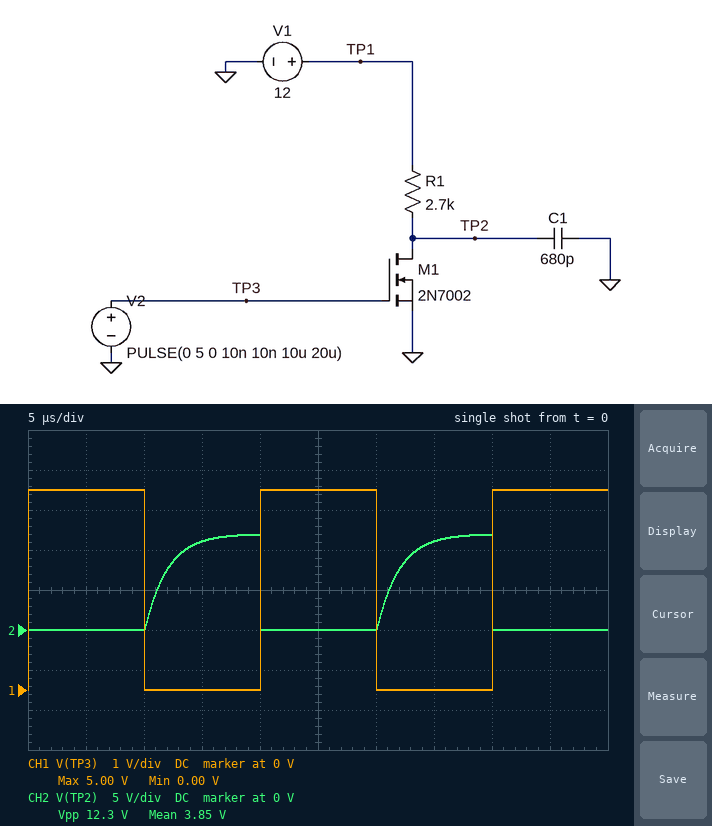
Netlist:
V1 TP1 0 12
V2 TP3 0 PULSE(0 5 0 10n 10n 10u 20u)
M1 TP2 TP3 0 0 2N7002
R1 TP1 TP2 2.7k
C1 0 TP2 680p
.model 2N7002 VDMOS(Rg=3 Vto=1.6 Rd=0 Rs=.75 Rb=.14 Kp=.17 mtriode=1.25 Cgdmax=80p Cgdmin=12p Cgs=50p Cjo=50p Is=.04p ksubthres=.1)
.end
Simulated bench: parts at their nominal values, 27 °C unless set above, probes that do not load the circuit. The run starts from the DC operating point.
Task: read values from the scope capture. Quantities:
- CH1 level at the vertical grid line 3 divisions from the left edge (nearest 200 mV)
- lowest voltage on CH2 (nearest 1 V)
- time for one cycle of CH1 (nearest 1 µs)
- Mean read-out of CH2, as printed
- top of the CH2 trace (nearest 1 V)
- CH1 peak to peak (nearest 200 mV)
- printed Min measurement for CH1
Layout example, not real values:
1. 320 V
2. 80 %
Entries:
1. 0 V
2. 0 V
3. 20 µs
4. 3.85 V
5. 12 V
6. 5.0 V
7. 0.00 V
